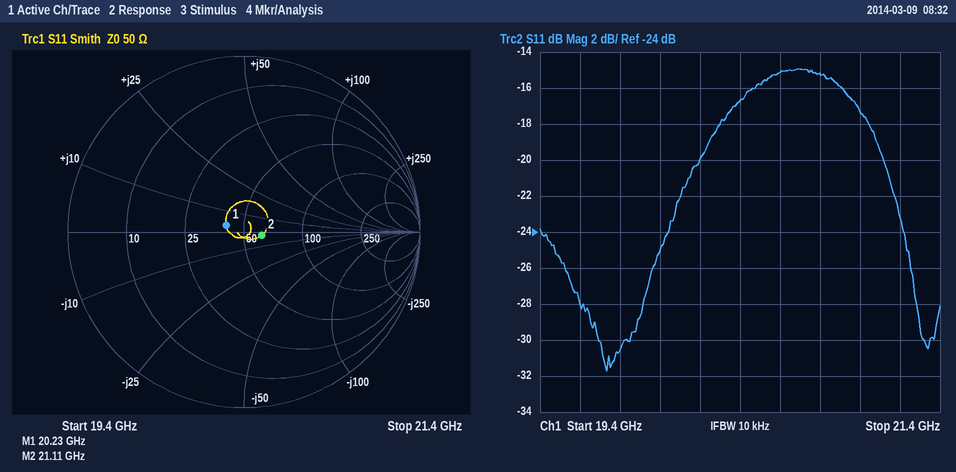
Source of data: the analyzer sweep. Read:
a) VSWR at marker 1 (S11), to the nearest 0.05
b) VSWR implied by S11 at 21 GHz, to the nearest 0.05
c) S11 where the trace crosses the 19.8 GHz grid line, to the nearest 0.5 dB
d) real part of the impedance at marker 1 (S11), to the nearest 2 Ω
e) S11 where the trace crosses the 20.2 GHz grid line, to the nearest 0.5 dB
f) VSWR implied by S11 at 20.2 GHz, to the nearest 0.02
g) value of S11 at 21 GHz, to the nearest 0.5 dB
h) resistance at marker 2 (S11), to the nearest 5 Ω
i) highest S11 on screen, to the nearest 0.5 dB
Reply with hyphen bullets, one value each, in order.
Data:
- 1.25
- 1.30
- -30.5 dB
- 40 Ω
- -20.0 dB
- 1.22
- -17.5 dB
- 60 Ω
- -15.0 dB
